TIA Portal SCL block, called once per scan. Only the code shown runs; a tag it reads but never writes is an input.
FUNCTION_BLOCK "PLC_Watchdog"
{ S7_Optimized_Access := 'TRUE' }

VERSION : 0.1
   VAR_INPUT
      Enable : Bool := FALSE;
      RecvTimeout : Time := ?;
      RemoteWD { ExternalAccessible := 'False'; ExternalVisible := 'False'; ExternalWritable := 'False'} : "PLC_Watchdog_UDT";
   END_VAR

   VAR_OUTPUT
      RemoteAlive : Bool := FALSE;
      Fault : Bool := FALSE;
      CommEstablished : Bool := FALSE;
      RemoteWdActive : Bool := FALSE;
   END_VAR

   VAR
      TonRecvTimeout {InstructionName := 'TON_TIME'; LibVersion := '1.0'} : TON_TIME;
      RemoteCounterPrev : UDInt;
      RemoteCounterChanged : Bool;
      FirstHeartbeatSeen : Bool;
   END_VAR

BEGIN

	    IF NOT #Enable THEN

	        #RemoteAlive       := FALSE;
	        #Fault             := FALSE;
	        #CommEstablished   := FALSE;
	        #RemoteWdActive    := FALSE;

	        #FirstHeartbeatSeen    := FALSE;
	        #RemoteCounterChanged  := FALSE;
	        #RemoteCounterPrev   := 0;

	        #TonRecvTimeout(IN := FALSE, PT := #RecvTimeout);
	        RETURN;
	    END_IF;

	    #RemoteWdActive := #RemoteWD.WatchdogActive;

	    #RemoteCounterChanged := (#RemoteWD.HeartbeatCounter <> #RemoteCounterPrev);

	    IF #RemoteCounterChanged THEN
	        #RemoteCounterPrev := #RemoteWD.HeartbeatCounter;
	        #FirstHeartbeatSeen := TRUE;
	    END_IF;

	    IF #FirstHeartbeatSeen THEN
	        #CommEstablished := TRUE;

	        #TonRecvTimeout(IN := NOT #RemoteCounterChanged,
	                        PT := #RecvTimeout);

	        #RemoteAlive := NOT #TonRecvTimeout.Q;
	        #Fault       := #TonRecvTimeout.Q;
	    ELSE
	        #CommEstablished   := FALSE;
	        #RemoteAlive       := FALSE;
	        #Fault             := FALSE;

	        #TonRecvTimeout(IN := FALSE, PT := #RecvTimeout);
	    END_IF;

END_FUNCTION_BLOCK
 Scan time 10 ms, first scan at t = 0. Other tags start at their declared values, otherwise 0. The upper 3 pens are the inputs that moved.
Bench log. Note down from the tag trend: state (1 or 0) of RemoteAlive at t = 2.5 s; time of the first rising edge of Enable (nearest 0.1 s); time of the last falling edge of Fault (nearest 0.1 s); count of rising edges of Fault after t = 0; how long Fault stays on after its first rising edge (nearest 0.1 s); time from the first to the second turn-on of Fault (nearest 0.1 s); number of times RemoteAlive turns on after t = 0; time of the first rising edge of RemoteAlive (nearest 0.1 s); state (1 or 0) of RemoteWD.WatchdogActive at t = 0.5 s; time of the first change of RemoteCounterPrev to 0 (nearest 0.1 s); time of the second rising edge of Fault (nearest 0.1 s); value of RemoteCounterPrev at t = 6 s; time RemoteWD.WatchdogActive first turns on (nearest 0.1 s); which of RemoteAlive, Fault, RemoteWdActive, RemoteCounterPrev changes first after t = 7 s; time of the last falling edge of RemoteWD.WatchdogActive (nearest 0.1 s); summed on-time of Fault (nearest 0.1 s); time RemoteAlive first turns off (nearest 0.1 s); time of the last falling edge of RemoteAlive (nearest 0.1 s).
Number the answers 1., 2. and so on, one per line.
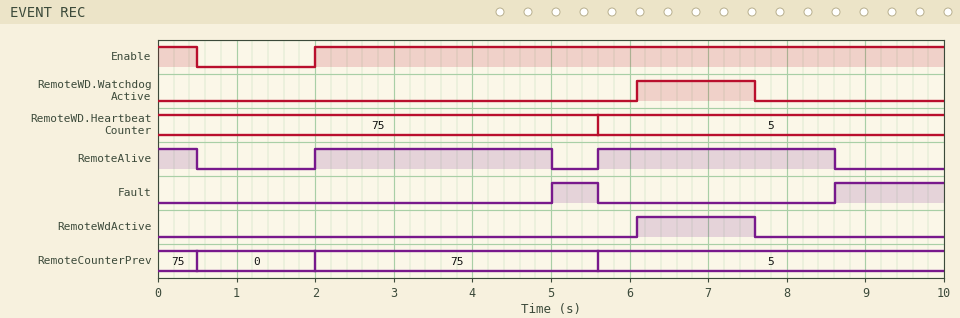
1. 1
2. 2.0 s
3. 5.6 s
4. 2
5. 0.6 s
6. 3.6 s
7. 2
8. 2.0 s
9. 0
10. 0.5 s
11. 8.6 s
12. 5
13. 6.1 s
14. RemoteWdActive
15. 7.6 s
16. 2.0 s
17. 0.5 s
18. 8.6 s
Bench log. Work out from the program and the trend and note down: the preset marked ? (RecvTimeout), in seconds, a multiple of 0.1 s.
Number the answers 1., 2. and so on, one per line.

1. 3.0 s
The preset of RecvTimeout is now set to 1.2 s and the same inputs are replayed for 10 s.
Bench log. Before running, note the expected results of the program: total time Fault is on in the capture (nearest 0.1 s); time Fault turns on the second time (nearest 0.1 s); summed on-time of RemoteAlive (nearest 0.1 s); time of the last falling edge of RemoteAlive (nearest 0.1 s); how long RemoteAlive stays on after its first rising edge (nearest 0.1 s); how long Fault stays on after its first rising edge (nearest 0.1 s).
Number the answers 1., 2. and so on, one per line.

1. 5.6 s
2. 6.8 s
3. 2.9 s
4. 6.8 s
5. 1.2 s
6. 2.4 s
